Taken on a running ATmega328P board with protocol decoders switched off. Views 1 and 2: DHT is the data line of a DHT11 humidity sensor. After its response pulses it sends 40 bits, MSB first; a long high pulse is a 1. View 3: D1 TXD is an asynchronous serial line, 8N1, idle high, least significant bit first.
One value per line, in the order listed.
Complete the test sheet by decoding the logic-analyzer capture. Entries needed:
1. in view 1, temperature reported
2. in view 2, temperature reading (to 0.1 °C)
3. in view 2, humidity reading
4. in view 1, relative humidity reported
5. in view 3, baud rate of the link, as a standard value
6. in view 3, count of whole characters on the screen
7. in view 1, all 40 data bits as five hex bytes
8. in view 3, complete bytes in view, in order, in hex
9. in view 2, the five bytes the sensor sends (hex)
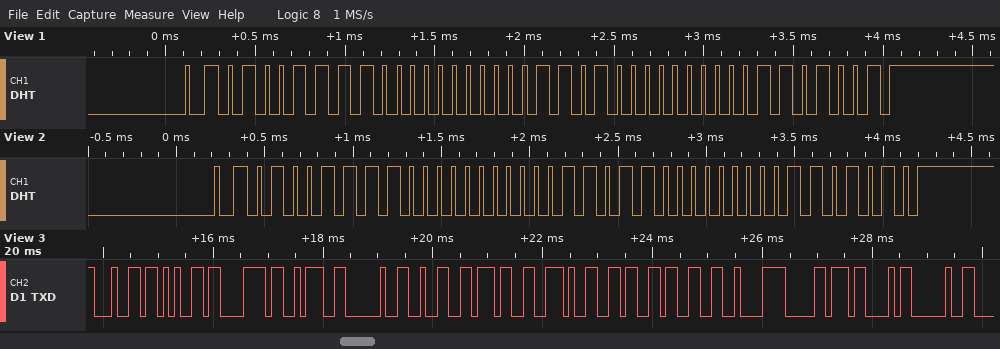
26.0 °C
27.0 °C
79 %
79 %
9600 baud
14
4F 00 1A 00 69
64 65 78 3A 20 32 37 2E 36 33 C2 B0 43 20
4F 00 1B 00 6A
